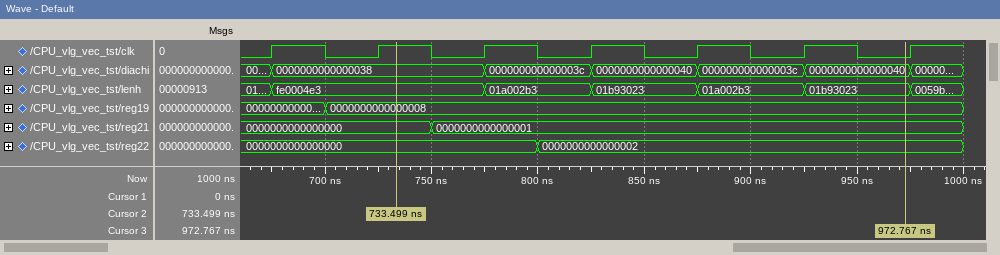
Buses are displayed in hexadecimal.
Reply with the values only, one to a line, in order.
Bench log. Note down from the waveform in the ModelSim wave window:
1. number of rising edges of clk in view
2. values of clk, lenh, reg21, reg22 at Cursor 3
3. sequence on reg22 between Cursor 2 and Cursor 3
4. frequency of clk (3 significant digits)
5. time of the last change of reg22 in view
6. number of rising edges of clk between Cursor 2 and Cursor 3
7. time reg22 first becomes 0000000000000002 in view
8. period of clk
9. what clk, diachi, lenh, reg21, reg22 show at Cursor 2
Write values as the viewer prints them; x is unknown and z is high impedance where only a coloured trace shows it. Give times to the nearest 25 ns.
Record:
7
clk=0, lenh=01b93023, reg21=0000000000000001, reg22=0000000000000002
0000000000000000, 0000000000000002
20.0 MHz
800 ns
4
800 ns
50 ns
clk=1, diachi=0000000000000038, lenh=fe0004e3, reg21=0000000000000000, reg22=0000000000000000
